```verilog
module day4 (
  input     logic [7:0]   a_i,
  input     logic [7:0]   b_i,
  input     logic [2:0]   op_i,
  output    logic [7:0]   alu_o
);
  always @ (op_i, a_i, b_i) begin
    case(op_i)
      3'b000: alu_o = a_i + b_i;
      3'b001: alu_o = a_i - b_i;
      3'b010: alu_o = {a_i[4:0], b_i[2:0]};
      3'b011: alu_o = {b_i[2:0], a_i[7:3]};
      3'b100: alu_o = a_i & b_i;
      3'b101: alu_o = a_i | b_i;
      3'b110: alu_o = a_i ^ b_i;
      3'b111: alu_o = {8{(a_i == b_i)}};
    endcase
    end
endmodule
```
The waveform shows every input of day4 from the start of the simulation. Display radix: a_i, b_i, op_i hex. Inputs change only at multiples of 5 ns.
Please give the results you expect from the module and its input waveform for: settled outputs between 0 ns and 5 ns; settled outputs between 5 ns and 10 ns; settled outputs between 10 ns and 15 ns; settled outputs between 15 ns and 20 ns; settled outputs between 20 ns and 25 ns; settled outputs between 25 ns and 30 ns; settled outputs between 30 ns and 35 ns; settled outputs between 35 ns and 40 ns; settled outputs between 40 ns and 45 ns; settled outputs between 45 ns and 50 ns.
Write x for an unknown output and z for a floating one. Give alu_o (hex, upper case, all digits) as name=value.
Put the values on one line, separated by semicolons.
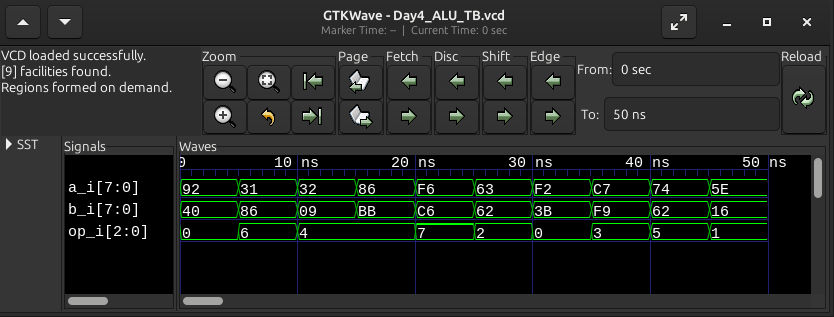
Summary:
alu_o=D2; alu_o=B7; alu_o=00; alu_o=82; alu_o=00; alu_o=1A; alu_o=2D; alu_o=38; alu_o=76; alu_o=48
